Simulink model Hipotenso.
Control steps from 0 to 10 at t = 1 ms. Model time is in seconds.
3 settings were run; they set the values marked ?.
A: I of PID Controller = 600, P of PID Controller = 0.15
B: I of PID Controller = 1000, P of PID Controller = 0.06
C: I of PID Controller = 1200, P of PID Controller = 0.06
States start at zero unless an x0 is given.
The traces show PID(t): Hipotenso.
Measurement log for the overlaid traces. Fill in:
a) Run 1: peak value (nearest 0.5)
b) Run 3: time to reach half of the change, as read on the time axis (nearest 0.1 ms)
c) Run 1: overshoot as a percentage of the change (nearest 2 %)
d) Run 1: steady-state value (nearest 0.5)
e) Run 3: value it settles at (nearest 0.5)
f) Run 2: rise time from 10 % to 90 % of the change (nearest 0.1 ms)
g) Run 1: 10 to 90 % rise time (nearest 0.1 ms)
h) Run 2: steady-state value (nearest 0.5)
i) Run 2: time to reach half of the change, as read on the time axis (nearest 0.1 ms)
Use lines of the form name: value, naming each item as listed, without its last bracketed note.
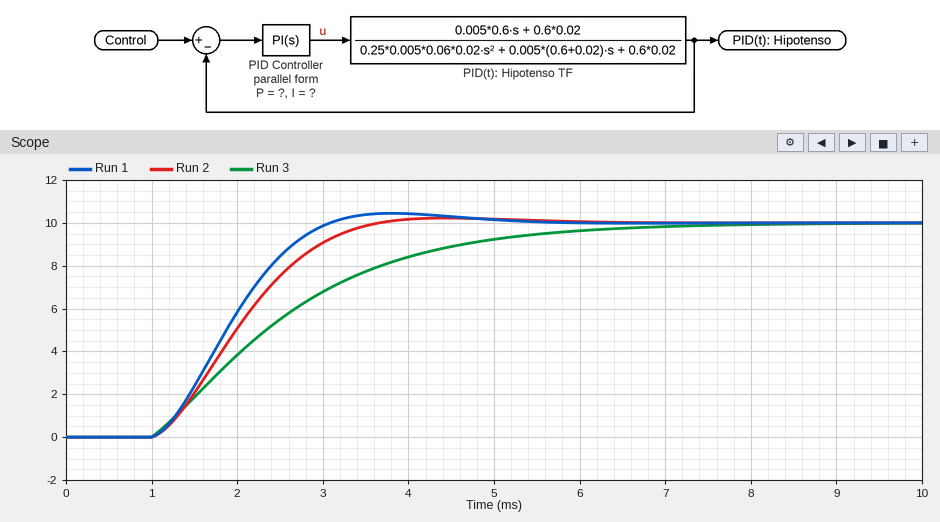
Run 1: peak value: 10.5
Run 3: time to reach half of the change, as read on the time axis: 2.3 ms
Run 1: overshoot as a percentage of the change: 4 %
Run 1: steady-state value: 10.0
Run 3: value it settles at: 10.0
Run 2: rise time from 10 % to 90 % of the change: 1.7 ms
Run 1: 10 to 90 % rise time: 1.4 ms
Run 2: steady-state value: 10.0
Run 2: time to reach half of the change, as read on the time axis: 2.0 ms
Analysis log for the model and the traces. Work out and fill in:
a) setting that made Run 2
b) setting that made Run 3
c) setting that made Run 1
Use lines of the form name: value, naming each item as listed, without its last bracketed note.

setting that made Run 2: B
setting that made Run 3: A
setting that made Run 1: C
